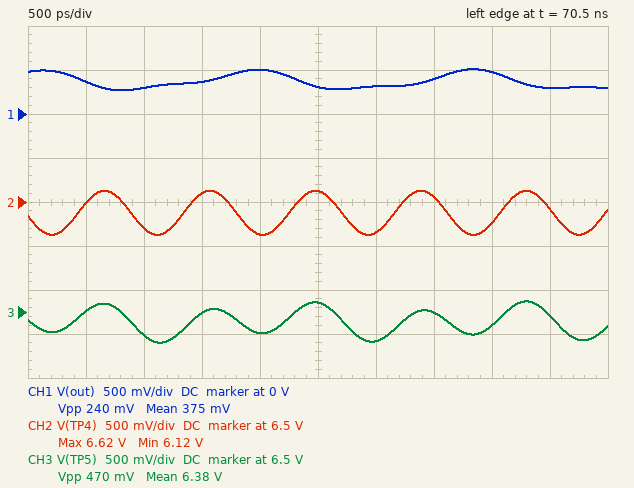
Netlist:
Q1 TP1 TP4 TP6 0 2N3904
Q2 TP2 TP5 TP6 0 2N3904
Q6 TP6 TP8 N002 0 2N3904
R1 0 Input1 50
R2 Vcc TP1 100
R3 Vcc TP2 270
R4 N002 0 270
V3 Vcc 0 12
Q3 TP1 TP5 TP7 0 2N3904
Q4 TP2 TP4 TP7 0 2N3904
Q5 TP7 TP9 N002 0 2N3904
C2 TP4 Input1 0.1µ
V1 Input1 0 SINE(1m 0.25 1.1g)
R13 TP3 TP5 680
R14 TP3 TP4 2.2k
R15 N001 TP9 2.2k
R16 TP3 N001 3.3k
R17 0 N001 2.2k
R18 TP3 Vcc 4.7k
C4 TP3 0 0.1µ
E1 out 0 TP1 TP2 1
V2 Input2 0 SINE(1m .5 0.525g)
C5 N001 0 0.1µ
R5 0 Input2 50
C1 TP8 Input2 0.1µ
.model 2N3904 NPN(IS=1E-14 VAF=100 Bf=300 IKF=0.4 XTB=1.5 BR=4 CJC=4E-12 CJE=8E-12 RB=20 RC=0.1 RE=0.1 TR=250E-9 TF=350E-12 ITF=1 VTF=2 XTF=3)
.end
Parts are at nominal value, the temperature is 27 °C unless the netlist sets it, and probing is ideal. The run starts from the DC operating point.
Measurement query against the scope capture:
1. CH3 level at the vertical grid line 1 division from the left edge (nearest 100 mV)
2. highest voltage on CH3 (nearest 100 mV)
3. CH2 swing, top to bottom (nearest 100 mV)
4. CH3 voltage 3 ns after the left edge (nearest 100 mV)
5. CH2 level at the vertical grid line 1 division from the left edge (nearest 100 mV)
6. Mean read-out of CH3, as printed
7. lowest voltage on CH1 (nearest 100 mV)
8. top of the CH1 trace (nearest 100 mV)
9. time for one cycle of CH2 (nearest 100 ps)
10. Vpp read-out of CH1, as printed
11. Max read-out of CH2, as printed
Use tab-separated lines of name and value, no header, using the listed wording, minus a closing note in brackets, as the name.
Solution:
CH3 level at the vertical grid line 1 division from the left edge	6.5 V
highest voltage on CH3	6.6 V
CH2 swing, top to bottom	500 mV
CH3 voltage 3 ns after the left edge	6.2 V
CH2 level at the vertical grid line 1 division from the left edge	6.5 V
Mean read-out of CH3, as printed	6.38 V
lowest voltage on CH1	300 mV
top of the CH1 trace	500 mV
time for one cycle of CH2	900 ps
Vpp read-out of CH1, as printed	240 mV
Max read-out of CH2, as printed	6.62 V
